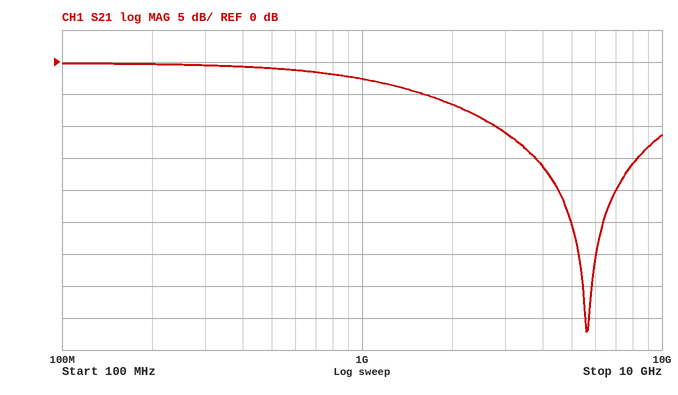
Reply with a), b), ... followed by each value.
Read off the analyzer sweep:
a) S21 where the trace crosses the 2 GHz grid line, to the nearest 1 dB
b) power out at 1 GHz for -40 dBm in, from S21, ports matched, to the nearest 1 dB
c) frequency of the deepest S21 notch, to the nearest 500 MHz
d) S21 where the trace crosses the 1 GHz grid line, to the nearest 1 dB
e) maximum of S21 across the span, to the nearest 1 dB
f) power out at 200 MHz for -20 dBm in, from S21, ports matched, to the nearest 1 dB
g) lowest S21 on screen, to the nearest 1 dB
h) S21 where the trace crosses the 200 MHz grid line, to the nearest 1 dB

a) -7 dB
b) -43 dBm
c) 5.5 GHz
d) -3 dB
e) 0 dB
f) -20 dBm
g) -42 dB
h) 0 dB
